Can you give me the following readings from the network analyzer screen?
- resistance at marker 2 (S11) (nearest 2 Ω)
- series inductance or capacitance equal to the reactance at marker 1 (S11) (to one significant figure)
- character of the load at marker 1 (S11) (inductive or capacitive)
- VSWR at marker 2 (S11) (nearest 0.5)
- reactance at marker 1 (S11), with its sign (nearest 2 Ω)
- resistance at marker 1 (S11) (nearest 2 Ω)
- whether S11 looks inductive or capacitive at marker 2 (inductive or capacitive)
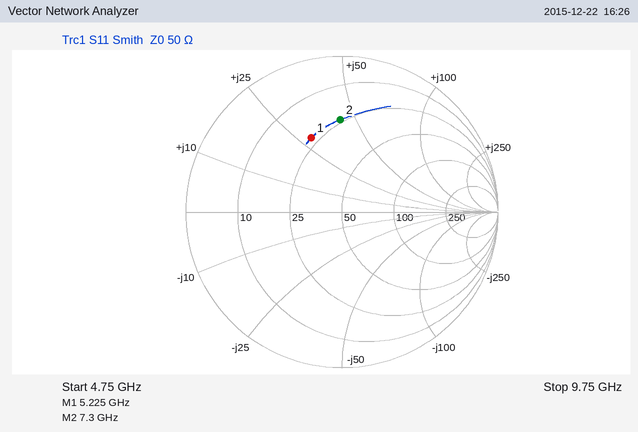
24 Ω
900 pH
inductive
4.0
+28 Ω
22 Ω
inductive
